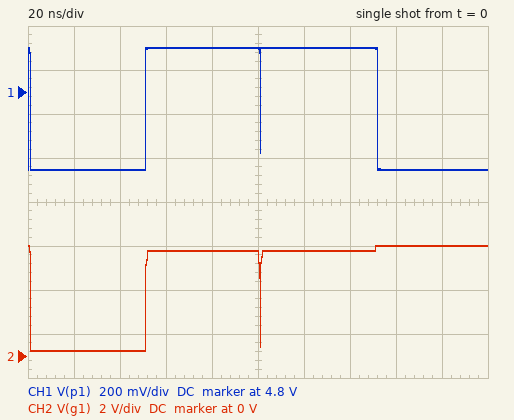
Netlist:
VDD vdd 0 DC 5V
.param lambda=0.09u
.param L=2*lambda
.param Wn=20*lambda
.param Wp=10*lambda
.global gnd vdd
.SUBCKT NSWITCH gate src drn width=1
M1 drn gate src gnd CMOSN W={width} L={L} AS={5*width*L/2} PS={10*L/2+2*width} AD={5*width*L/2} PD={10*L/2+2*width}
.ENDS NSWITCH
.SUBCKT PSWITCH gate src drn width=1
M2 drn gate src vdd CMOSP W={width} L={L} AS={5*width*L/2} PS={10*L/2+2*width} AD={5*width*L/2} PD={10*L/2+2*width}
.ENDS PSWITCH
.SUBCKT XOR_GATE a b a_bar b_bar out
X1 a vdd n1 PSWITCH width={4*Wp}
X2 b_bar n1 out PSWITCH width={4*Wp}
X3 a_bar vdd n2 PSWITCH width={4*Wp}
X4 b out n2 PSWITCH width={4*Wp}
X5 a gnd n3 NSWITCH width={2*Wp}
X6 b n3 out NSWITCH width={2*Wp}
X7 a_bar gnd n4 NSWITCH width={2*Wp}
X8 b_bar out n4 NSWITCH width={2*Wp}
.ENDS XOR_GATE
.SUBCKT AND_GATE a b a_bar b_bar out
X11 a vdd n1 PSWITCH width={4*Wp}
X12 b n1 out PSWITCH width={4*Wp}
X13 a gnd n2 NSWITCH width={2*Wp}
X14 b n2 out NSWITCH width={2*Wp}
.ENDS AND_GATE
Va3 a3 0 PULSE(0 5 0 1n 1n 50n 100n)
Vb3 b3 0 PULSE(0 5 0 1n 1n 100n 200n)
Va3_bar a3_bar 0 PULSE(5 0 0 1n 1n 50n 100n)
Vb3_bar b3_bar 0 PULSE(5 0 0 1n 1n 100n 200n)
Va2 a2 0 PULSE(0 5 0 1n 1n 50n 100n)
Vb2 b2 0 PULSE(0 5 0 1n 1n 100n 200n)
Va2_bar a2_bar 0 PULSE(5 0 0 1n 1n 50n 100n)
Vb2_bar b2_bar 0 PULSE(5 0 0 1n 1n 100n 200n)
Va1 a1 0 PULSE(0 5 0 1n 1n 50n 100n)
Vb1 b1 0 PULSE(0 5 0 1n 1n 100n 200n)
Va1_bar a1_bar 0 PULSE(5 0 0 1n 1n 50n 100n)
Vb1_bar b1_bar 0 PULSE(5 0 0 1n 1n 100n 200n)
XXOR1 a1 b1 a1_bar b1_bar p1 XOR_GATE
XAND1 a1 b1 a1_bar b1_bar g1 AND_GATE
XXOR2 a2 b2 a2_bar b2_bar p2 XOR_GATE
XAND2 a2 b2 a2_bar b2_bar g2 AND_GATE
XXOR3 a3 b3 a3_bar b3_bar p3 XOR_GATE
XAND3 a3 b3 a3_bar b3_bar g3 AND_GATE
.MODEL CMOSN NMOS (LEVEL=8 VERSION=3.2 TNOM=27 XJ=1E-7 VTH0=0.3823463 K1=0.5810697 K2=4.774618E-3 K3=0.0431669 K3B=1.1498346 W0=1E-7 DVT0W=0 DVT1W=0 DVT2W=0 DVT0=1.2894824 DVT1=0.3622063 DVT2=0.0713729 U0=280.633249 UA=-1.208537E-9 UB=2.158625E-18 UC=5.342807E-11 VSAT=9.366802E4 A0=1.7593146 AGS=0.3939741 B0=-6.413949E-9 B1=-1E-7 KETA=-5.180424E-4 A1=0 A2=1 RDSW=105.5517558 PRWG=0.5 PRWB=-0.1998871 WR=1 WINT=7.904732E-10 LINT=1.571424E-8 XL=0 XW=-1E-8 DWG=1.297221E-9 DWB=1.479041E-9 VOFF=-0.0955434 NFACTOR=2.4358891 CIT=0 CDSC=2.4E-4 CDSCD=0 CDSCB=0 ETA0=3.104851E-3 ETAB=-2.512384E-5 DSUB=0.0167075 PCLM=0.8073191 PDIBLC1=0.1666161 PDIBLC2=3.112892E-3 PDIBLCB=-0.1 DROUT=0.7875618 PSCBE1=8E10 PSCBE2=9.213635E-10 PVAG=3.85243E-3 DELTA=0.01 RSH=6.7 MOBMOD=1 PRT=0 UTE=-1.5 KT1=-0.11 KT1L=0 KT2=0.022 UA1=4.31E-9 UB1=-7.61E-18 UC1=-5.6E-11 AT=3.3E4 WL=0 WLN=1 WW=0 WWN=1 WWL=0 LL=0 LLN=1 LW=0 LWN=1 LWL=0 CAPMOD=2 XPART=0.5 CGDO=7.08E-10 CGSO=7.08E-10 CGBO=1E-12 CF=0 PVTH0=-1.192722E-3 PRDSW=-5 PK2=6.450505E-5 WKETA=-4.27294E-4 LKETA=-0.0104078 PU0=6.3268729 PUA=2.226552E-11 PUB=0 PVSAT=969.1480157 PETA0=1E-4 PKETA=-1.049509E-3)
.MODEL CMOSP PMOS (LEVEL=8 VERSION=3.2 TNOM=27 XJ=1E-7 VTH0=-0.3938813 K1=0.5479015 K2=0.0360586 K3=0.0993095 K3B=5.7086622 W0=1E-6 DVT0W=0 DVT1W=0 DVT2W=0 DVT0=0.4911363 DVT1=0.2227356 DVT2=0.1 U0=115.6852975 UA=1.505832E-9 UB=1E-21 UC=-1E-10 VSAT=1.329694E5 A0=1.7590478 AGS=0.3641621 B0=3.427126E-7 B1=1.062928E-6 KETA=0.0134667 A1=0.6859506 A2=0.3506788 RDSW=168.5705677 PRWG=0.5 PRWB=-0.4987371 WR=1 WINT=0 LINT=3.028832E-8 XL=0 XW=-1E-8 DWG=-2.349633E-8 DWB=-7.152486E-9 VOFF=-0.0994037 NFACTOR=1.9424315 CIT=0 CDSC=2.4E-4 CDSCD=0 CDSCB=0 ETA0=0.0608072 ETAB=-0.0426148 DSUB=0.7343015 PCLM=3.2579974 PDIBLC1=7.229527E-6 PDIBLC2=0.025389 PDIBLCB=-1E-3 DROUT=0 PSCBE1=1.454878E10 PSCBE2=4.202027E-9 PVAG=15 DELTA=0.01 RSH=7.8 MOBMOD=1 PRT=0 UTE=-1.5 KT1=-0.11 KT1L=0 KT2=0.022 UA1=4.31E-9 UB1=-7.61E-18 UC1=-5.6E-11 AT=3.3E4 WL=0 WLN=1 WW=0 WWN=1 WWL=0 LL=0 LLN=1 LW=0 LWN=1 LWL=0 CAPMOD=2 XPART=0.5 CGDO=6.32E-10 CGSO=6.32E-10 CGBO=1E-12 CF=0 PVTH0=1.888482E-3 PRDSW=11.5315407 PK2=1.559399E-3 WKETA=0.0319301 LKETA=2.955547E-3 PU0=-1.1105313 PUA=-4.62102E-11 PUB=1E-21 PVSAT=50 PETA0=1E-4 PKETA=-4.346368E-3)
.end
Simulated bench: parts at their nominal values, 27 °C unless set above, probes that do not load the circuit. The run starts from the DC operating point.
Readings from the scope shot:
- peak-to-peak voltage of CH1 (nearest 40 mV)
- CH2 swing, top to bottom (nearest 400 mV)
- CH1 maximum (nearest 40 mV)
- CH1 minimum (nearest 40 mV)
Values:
560 mV
4.8 V
5.00 V
4.44 V
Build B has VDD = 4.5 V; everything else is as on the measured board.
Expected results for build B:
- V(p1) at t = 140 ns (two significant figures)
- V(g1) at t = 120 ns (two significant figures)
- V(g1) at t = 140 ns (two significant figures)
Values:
4.5 V
360 mV
380 mV
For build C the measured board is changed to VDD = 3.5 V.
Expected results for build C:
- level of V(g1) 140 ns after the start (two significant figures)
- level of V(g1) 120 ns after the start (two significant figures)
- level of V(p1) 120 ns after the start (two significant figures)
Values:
360 mV
350 mV
3.5 V
